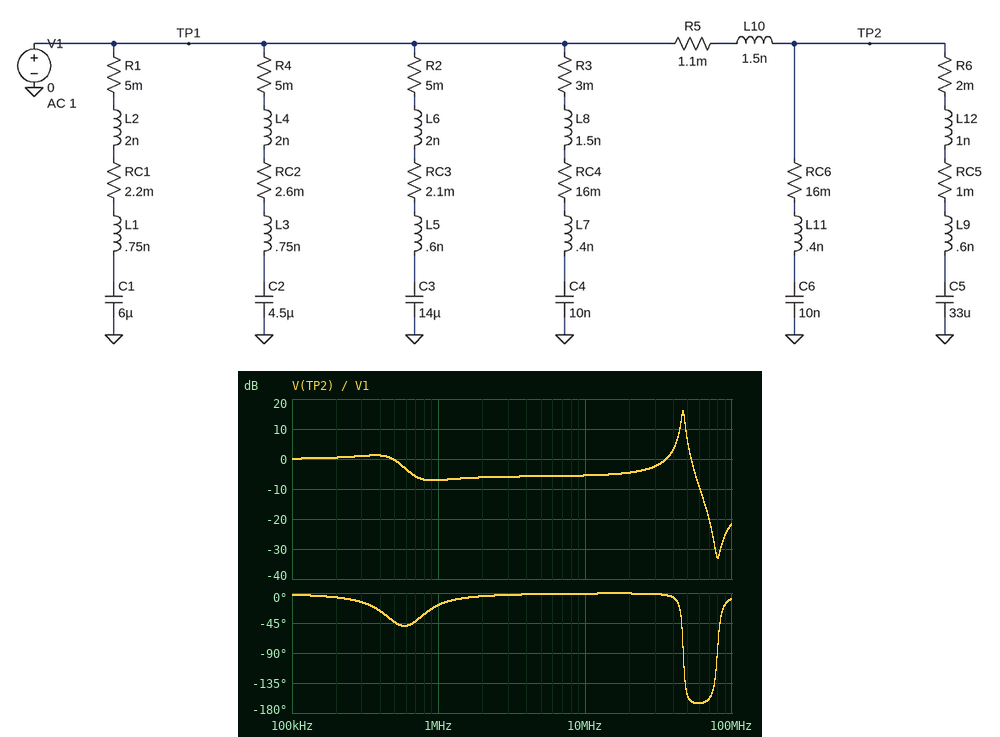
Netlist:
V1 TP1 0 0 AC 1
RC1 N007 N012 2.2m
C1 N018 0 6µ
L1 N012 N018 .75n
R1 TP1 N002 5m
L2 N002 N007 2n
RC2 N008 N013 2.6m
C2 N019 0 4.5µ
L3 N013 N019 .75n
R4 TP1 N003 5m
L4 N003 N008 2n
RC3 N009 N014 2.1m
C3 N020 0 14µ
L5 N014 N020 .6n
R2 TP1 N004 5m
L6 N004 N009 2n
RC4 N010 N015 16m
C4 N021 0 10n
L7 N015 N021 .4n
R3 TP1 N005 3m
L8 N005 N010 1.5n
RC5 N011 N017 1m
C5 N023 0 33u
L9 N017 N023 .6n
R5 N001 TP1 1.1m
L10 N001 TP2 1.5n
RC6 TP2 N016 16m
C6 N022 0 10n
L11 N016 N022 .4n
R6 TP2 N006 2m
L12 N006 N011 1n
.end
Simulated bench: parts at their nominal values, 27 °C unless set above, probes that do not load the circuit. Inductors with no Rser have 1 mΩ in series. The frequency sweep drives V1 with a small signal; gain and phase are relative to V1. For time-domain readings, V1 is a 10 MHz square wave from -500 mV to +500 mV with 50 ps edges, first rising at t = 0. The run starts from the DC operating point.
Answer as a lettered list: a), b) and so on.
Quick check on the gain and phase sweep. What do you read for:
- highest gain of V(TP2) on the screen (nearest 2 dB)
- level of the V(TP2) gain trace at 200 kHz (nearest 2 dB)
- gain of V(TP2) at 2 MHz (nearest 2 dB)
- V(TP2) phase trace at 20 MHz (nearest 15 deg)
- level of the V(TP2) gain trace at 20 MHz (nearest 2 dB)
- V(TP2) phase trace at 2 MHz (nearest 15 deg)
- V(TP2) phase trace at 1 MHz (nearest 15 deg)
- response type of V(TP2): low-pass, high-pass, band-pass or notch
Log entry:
a) 16 dB
b) 0 dB
c) -6 dB
d) 0 deg
e) -4 dB
f) 0 deg
g) -15 deg
h) band-pass
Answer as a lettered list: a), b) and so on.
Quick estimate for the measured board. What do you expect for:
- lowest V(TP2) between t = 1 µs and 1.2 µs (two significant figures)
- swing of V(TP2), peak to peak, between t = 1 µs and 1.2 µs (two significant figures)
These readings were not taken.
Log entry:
a) -520 mV
b) 1.2 V
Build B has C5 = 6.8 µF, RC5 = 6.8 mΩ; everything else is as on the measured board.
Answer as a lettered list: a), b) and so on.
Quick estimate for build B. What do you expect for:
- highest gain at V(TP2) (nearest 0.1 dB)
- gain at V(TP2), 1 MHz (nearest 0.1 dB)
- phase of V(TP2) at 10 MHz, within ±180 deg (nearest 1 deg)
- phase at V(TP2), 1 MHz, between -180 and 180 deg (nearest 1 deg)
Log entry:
a) 15.3 dB
b) 2.1 dB
c) -3 deg
d) -34 deg
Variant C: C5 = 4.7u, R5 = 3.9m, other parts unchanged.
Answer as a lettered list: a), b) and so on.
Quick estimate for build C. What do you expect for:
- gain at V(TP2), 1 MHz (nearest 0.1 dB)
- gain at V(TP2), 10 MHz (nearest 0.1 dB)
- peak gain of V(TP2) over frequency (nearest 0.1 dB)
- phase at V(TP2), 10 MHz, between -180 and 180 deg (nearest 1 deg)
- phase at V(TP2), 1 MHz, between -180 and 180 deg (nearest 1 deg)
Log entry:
a) 2.9 dB
b) -5.6 dB
c) 15.6 dB
d) 0 deg
e) -23 deg
